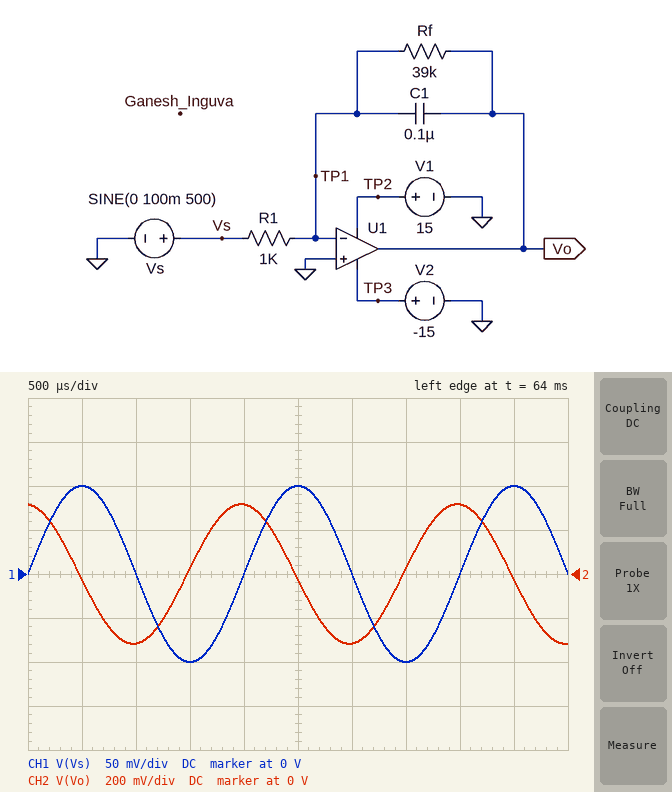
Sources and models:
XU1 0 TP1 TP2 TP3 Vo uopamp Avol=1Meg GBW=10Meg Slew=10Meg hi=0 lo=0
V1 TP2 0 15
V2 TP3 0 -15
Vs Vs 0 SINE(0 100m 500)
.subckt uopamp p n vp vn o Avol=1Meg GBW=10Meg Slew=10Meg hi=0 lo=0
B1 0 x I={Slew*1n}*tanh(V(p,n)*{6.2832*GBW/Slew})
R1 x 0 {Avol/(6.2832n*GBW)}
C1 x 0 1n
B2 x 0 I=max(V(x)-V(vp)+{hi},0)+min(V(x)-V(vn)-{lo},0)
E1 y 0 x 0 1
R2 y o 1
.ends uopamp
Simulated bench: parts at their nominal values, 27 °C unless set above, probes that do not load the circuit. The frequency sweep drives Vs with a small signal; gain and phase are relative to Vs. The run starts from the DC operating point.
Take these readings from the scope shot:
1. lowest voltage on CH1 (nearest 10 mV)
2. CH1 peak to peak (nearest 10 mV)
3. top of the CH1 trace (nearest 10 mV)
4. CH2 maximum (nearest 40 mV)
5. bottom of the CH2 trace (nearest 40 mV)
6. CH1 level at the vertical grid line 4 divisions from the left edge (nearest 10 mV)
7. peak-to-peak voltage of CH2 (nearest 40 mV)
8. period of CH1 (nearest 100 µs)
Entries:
-100 mV
200 mV
100 mV
320 mV
-320 mV
0 V
640 mV
2.0 ms
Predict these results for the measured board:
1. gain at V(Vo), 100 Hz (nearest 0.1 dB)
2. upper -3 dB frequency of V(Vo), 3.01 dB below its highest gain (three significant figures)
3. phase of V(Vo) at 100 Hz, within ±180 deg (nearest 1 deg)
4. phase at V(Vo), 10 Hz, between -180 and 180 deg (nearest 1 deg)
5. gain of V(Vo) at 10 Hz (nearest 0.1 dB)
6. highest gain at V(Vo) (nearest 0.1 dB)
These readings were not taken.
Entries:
23.4 dB
40.8 Hz
112 deg
166 deg
31.6 dB
31.8 dB
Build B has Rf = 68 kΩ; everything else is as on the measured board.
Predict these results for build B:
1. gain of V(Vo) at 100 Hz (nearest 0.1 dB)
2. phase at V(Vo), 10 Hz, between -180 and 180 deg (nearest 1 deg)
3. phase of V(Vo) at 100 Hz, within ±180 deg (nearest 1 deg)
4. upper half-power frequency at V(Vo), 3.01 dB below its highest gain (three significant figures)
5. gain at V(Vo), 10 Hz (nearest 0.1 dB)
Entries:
23.8 dB
157 deg
103 deg
23.4 Hz
35.9 dB
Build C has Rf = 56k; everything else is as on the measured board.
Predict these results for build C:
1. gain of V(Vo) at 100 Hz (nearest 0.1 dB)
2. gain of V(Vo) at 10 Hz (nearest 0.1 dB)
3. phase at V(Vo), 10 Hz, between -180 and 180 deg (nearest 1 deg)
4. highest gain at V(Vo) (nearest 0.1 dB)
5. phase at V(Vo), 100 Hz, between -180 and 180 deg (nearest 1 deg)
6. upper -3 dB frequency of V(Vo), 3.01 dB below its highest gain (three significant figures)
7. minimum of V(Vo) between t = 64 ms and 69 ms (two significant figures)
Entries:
23.7 dB
34.5 dB
161 deg
35.0 dB
106 deg
28.4 Hz
-320 mV
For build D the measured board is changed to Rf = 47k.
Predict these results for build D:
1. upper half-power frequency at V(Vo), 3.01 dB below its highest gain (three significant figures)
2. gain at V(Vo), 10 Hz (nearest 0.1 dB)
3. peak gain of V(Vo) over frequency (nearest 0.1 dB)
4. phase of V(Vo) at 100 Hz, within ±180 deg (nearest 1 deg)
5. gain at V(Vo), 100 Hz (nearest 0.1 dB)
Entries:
33.9 Hz
33.1 dB
33.4 dB
109 deg
23.6 dB
